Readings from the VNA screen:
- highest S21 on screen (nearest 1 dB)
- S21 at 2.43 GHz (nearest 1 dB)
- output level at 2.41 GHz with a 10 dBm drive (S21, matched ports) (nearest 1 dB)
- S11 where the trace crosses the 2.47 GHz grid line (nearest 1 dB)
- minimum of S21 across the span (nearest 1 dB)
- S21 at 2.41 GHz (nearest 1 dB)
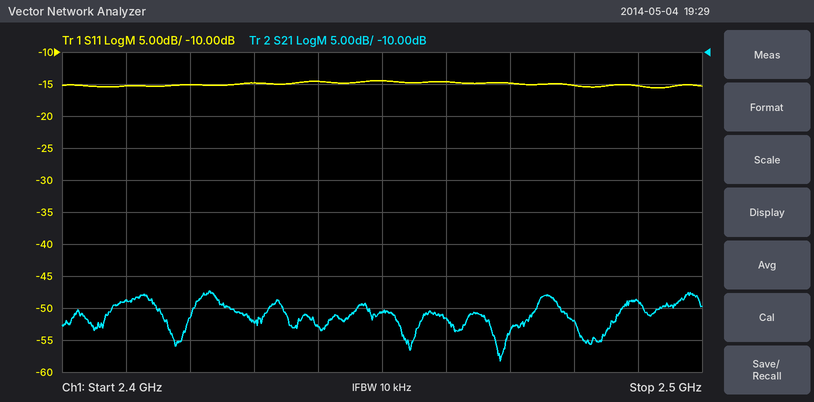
-47 dB
-52 dB
-39 dBm
-15 dB
-58 dB
-49 dB
